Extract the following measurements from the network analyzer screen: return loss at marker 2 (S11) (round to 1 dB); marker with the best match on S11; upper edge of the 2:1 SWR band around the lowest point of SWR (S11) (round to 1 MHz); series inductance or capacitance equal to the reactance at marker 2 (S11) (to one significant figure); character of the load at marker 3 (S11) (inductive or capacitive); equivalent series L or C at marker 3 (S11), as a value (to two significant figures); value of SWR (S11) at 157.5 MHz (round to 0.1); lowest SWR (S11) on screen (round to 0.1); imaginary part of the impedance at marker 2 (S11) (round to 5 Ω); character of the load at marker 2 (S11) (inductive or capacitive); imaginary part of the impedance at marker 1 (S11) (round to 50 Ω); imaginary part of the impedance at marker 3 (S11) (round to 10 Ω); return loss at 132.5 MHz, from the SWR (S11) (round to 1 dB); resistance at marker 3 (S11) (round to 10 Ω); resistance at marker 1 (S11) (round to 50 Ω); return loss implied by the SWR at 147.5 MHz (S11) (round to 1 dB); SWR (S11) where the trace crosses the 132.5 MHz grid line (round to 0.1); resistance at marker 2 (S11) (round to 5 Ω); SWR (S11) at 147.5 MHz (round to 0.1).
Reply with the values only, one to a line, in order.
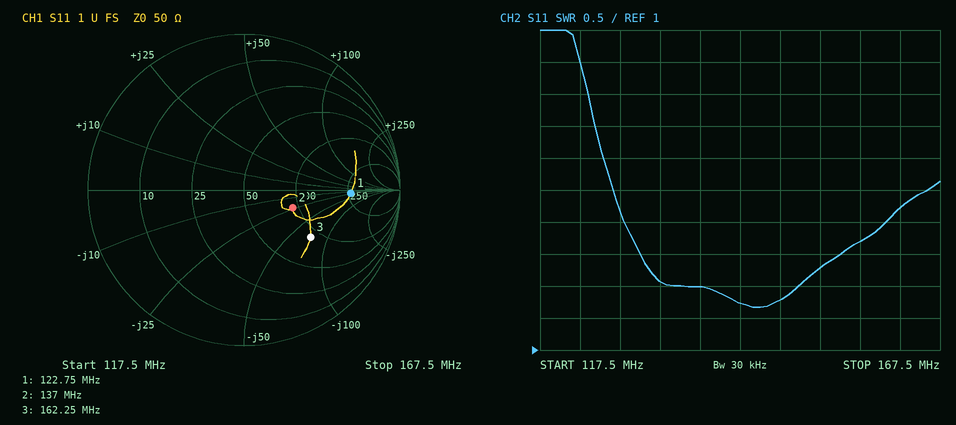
10 dB
marker 2
150 MHz
50 pF
capacitive
14 pF
2.7
1.7
-25 Ω
capacitive
0 Ω
-70 Ω
9 dB
90 Ω
250 Ω
11 dB
2.1
90 Ω
1.8
